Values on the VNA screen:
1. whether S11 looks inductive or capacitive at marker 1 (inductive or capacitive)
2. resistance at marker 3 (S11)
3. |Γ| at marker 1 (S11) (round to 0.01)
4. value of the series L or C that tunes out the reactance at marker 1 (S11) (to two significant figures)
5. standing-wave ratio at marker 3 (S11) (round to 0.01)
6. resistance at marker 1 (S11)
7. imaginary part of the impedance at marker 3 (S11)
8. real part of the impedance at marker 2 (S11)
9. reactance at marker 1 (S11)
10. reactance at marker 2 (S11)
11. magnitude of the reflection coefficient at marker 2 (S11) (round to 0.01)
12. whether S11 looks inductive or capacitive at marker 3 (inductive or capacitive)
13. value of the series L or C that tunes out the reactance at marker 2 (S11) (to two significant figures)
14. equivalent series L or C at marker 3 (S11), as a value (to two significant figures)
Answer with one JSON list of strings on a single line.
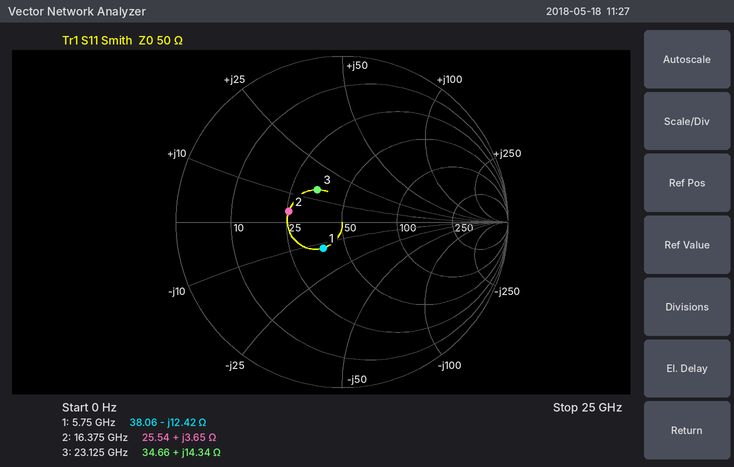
["capacitive", "34.66 Ω", "0.19", "340 pH", "1.65", "38.06 Ω", "+14.34 Ω", "25.54 Ω", "-12.42 Ω", "+3.65 Ω", "0.33", "inductive", "2.7 pF", "99 pH"]
